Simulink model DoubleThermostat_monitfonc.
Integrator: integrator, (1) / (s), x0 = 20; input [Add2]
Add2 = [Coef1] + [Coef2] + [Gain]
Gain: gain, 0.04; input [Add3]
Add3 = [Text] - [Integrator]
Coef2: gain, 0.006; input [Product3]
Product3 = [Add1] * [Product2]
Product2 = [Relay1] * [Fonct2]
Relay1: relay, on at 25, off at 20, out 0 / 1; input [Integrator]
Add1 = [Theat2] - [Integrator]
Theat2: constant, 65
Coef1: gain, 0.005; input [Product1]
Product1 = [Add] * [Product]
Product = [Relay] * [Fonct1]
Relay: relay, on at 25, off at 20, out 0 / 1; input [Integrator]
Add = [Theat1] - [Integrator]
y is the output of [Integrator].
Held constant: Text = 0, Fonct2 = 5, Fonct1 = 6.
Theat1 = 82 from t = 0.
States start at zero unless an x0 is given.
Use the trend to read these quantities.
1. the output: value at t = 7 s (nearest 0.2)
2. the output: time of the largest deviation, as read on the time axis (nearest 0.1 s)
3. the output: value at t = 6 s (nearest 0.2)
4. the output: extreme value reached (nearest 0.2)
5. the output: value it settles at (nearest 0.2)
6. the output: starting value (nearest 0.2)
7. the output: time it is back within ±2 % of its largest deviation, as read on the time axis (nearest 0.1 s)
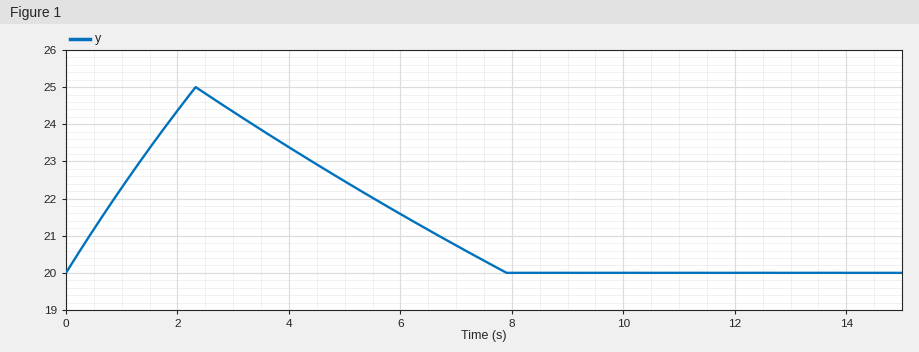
20.8
2.3 s
21.6
25.0
20.0
20.0
7.8 s
